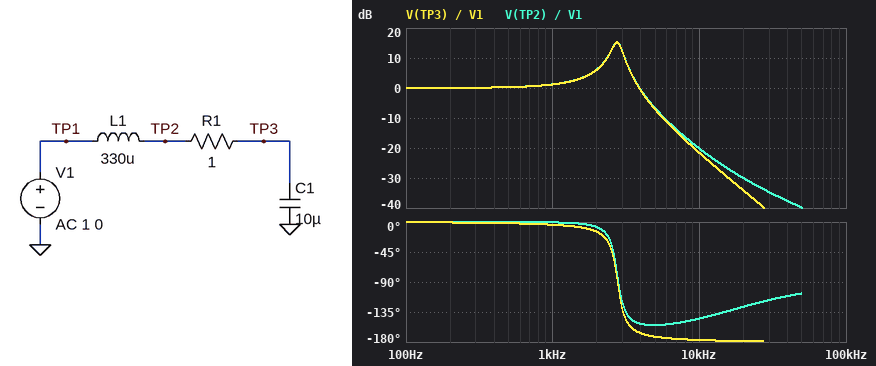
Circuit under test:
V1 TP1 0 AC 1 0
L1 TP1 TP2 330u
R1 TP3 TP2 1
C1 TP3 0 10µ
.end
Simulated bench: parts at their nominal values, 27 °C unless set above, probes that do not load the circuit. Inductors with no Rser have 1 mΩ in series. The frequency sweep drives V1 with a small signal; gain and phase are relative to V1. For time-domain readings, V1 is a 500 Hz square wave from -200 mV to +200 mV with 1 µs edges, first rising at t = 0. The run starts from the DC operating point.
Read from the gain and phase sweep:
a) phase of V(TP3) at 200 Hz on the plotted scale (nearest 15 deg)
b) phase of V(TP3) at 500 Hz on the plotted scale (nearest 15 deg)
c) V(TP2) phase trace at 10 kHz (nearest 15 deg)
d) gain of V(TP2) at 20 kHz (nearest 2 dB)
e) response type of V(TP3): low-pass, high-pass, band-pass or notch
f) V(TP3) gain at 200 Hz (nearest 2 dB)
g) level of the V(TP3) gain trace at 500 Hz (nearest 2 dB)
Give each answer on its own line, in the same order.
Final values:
0 deg
0 deg
-150 deg
-30 dB
low-pass
0 dB
0 dB
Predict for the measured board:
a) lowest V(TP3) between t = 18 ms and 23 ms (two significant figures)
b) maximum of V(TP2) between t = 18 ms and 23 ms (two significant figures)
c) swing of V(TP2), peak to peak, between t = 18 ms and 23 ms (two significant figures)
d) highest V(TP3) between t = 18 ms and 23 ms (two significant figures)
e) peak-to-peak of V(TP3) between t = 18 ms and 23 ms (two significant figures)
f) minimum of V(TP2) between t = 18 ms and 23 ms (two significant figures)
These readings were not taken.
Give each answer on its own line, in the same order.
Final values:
-500 mV
500 mV
1.0 V
500 mV
1.0 V
-500 mV
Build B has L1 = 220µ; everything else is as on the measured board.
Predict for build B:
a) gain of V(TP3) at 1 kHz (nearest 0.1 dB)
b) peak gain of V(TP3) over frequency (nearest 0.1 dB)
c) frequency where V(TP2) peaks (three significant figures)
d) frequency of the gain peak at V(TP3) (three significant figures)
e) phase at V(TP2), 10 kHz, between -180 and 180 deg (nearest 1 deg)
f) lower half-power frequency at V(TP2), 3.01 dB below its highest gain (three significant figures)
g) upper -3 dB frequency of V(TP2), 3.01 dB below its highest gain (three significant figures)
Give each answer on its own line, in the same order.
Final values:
0.8 dB
13.5 dB
3.36 kHz
3.35 kHz
-143 deg
2.97 kHz
3.70 kHz
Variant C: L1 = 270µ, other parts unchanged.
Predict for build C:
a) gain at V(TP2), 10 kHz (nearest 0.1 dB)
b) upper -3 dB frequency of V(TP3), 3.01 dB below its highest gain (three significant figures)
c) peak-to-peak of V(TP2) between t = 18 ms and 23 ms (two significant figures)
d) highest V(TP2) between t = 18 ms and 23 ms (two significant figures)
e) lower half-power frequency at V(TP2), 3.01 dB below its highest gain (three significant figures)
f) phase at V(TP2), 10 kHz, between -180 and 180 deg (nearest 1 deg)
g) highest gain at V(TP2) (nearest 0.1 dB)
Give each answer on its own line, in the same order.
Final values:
-18.3 dB
3.32 kHz
920 mV
460 mV
2.72 kHz
-144 deg
14.5 dB
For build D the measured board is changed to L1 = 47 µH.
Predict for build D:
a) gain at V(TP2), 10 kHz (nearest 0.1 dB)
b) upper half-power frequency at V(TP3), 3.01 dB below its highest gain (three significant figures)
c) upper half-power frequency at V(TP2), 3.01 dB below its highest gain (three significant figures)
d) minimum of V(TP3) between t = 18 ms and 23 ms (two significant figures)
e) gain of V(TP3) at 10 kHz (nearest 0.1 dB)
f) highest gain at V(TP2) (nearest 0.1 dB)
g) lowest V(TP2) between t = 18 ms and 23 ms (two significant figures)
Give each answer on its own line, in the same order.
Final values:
0.9 dB
8.51 kHz
8.62 kHz
-390 mV
-0.5 dB
7.7 dB
-410 mV
